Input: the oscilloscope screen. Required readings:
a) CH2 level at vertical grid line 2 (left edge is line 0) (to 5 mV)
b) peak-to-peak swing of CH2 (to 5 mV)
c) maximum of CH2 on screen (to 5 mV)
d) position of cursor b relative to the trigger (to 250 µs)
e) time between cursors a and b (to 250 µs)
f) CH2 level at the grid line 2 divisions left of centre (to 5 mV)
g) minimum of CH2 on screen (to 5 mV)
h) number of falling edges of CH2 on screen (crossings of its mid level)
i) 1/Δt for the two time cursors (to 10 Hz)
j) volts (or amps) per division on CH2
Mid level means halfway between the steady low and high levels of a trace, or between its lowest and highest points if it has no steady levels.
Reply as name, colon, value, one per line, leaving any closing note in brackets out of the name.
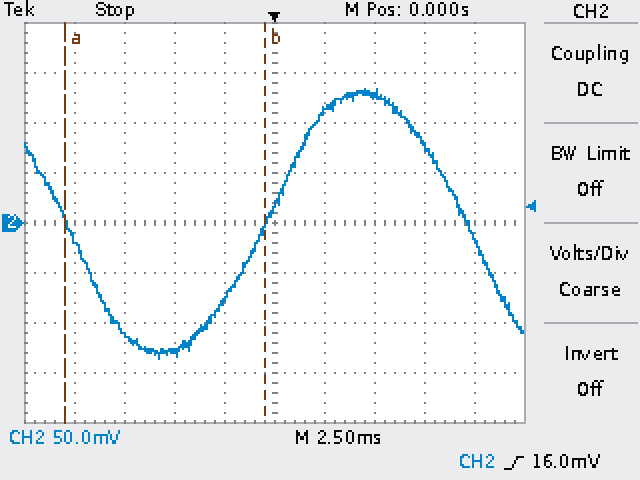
CH2 level at vertical grid line 2 (left edge is line 0): -110 mV
peak-to-peak swing of CH2: 270 mV
maximum of CH2 on screen: 135 mV
position of cursor b relative to the trigger: -500 µs
time between cursors a and b: 10.00 ms
CH2 level at the grid line 2 divisions left of centre: -130 mV
minimum of CH2 on screen: -135 mV
number of falling edges of CH2 on screen: 2
1/Δt for the two time cursors: 100 Hz
volts (or amps) per division on CH2: 50 mV
